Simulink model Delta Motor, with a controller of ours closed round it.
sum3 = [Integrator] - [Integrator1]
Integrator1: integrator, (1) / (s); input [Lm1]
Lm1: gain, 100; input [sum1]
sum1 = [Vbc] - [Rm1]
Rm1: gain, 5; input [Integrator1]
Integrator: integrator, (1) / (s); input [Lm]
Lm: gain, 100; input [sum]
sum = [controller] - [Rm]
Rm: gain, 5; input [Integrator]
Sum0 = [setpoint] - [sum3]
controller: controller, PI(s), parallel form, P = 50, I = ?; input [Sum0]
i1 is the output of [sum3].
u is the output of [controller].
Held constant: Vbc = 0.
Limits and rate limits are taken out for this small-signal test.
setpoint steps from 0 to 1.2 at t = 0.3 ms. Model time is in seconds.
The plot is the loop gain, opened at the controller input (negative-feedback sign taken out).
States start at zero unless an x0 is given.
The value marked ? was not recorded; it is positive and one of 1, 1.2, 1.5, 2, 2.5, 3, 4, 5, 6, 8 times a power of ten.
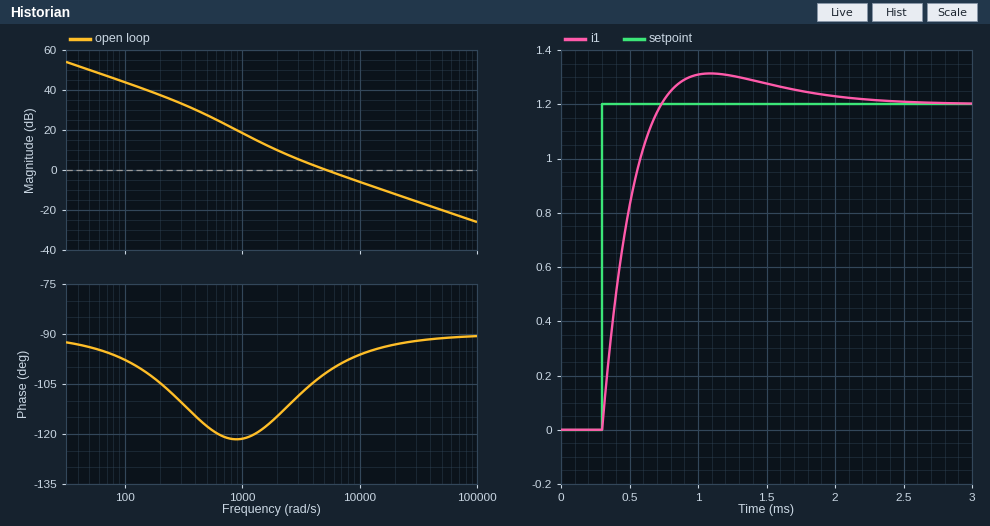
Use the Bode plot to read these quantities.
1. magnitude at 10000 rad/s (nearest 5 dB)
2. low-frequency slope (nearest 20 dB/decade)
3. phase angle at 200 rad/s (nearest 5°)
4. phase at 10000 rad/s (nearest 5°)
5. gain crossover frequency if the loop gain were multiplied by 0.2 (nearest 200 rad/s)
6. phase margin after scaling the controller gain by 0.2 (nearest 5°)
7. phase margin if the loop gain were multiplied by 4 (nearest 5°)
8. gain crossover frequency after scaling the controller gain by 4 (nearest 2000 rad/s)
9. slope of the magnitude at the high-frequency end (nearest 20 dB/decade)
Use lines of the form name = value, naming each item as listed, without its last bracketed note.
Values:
magnitude at 10000 rad/s = -5 dB
low-frequency slope = -20 dB/decade
phase angle at 200 rad/s = -105°
phase at 10000 rad/s = -95°
gain crossover frequency if the loop gain were multiplied by 0.2 = 1400 rad/s
phase margin after scaling the controller gain by 0.2 = 60°
phase margin if the loop gain were multiplied by 4 = 85°
gain crossover frequency after scaling the controller gain by 4 = 20000 rad/s
slope of the magnitude at the high-frequency end = -20 dB/decade
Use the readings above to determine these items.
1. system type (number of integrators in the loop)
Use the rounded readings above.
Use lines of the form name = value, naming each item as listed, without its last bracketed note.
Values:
system type = 1
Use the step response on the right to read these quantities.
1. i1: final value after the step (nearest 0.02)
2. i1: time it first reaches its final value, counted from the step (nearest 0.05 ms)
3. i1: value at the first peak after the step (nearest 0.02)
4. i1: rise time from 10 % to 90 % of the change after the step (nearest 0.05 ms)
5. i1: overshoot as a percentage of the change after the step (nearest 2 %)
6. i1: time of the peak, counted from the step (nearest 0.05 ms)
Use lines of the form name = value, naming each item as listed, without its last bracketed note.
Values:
i1: final value after the step = 1.20
i1: time it first reaches its final value, counted from the step = 0.45 ms
i1: value at the first peak after the step = 1.32
i1: rise time from 10 % to 90 % of the change after the step = 0.30 ms
i1: overshoot as a percentage of the change after the step = 10 %
i1: time of the peak, counted from the step = 0.80 ms
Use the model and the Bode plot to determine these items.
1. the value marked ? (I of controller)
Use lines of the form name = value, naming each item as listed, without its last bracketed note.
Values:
the value marked ? = 80000
